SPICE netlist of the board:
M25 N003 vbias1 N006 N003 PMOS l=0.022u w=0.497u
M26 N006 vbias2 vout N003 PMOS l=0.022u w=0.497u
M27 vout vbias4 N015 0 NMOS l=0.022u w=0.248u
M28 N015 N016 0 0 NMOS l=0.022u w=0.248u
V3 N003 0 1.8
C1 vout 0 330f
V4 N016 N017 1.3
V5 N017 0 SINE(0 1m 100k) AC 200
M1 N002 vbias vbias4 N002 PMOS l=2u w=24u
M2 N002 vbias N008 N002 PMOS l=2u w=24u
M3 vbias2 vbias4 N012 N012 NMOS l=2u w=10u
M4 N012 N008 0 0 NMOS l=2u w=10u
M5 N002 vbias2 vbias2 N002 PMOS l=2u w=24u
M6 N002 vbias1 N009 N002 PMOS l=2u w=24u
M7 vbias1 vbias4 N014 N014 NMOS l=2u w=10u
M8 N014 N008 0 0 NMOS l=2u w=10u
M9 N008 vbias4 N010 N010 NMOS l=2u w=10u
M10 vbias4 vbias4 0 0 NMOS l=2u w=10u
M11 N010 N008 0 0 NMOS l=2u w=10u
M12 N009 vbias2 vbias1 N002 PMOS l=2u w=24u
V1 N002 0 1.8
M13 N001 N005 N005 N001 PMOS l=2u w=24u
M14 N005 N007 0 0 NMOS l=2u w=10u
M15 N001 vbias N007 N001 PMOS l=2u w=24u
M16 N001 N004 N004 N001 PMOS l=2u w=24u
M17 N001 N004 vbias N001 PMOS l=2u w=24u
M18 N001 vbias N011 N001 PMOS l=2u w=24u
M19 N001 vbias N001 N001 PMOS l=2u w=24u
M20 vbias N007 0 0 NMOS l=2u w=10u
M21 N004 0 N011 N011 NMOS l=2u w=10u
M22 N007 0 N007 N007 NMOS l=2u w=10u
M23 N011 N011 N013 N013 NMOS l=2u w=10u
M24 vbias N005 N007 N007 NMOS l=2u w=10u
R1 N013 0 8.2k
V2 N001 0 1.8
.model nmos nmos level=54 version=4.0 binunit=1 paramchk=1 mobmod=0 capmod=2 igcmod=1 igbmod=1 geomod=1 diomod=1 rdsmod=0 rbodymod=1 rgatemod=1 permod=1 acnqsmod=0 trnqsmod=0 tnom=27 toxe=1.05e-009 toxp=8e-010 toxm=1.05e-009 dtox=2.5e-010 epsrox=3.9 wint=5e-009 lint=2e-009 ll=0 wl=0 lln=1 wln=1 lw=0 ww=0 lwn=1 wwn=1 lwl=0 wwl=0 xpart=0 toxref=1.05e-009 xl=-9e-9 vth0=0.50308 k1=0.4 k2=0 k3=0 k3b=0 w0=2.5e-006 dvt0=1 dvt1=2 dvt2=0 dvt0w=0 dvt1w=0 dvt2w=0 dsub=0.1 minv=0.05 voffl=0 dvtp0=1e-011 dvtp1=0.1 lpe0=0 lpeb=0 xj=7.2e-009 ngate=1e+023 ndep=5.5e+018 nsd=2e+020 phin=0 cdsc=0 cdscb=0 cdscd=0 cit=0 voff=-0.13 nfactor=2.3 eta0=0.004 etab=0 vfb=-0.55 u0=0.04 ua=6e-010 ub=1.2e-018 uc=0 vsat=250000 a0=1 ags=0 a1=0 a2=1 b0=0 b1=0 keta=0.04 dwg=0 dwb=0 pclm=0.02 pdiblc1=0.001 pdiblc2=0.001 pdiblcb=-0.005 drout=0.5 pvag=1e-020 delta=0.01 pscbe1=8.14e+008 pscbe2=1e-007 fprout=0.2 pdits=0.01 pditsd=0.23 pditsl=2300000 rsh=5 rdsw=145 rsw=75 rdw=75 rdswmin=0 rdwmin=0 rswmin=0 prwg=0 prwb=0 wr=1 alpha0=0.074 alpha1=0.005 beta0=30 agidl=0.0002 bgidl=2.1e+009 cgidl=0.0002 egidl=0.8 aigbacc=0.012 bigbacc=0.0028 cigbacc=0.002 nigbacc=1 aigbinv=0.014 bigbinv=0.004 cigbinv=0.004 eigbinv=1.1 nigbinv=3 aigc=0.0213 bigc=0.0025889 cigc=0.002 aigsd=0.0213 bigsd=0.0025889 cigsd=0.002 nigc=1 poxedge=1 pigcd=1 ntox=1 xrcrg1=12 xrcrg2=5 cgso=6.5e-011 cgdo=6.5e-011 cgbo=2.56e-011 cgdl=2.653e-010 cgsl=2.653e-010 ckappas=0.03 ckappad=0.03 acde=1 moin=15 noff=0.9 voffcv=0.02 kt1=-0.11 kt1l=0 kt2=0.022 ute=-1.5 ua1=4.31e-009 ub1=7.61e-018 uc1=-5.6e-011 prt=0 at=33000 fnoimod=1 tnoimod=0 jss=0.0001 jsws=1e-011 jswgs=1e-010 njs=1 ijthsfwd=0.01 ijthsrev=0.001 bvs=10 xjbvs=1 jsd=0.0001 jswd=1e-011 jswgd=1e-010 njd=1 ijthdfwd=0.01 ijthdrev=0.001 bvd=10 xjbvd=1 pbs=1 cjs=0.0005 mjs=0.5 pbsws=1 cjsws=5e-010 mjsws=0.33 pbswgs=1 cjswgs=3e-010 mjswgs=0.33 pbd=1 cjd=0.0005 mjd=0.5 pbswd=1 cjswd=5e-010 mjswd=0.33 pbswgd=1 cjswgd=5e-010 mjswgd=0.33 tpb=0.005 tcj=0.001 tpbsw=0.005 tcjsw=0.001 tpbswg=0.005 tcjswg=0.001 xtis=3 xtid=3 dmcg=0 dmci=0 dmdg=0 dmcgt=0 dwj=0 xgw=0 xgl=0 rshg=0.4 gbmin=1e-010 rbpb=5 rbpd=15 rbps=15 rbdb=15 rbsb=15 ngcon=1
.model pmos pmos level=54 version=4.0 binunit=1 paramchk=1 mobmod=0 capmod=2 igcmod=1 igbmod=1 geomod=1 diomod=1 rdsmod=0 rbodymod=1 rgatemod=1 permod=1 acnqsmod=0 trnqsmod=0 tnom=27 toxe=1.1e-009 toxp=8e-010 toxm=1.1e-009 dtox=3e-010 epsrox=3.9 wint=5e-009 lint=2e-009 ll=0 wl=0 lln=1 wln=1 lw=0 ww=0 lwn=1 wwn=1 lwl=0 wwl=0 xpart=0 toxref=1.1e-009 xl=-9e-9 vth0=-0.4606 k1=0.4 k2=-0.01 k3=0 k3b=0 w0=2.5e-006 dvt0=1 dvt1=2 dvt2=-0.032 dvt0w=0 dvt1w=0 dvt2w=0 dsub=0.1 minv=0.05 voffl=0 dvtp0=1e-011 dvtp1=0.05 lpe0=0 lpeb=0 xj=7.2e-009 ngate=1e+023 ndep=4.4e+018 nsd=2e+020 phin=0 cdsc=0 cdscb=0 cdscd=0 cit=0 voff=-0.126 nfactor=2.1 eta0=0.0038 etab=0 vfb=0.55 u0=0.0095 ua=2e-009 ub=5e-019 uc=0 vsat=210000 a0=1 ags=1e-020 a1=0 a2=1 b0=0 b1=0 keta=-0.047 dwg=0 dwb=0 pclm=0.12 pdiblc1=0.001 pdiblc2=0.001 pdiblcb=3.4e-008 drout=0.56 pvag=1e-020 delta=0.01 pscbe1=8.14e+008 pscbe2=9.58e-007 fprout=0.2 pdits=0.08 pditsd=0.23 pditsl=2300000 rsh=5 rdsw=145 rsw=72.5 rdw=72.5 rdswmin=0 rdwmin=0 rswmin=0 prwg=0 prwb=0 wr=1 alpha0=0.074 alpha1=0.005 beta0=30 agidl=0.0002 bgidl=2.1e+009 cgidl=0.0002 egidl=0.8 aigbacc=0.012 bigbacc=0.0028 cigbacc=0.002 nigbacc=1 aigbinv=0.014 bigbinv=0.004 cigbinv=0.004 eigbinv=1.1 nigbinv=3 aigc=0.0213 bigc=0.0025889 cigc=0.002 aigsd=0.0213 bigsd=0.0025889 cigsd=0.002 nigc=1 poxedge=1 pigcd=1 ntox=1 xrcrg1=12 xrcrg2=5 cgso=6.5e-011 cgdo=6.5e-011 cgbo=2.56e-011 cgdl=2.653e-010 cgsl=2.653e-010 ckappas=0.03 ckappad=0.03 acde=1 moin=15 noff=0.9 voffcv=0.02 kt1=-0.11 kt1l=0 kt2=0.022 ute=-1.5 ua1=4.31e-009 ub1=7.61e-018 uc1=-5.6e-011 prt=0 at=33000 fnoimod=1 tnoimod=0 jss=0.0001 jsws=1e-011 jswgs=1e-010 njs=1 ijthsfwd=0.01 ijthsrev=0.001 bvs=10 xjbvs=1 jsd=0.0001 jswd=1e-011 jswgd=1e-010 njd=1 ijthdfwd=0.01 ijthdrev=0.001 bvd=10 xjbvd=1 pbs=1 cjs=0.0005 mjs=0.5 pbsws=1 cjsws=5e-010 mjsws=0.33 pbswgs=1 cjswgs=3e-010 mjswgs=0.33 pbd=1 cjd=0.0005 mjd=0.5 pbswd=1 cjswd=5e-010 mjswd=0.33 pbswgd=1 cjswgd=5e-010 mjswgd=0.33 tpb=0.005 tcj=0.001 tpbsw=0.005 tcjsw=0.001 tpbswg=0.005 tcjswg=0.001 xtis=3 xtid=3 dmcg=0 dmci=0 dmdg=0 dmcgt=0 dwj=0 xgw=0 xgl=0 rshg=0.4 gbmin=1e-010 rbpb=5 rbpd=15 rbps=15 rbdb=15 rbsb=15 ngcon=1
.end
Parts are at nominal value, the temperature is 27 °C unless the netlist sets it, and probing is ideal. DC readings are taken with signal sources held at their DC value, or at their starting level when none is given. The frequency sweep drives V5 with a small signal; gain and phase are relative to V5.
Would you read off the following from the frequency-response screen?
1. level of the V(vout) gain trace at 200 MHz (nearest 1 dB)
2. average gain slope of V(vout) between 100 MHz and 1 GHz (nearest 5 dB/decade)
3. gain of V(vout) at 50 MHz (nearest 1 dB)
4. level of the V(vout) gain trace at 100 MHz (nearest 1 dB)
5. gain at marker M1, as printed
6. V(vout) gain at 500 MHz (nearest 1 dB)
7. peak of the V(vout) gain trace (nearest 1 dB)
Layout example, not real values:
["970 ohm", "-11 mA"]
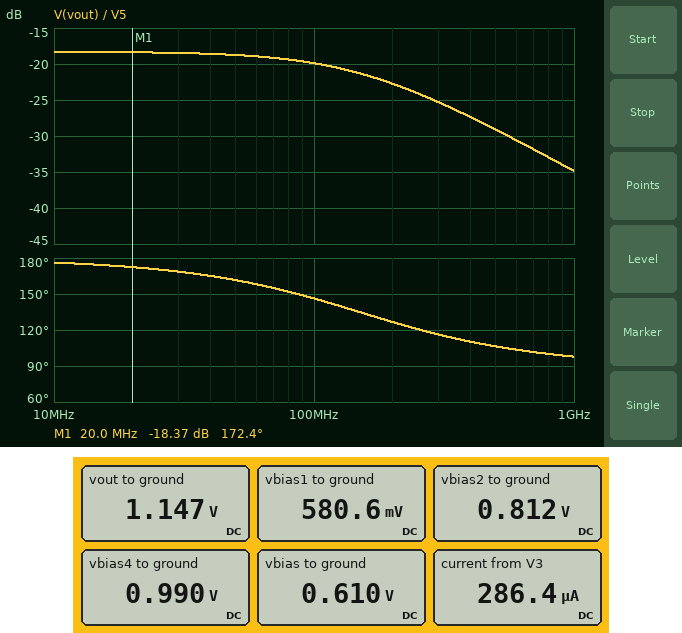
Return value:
["-23 dB", "-15 dB/decade", "-19 dB", "-20 dB", "-18.37 dB", "-29 dB", "-18 dB"]
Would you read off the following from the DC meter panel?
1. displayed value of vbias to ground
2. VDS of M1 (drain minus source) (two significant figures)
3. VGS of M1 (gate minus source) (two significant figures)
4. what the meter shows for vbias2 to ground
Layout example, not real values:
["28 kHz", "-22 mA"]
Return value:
["0.610 V", "810 mV", "-380 mV", "0.812 V"]
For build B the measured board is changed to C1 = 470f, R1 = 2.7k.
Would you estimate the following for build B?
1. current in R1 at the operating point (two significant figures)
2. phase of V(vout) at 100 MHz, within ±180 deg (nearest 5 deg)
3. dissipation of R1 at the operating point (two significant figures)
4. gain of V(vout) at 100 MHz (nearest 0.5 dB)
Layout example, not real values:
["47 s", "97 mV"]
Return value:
["63 µA", "135 deg", "11 µW", "-21.0 dB"]
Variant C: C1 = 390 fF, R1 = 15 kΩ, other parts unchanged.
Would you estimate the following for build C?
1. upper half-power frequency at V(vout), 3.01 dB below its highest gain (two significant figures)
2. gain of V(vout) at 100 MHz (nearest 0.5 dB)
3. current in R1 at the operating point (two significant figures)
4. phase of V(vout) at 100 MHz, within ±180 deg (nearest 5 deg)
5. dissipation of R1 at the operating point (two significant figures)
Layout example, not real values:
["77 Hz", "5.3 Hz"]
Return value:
["130 MHz", "-20.5 dB", "21 µA", "140 deg", "6.8 µW"]
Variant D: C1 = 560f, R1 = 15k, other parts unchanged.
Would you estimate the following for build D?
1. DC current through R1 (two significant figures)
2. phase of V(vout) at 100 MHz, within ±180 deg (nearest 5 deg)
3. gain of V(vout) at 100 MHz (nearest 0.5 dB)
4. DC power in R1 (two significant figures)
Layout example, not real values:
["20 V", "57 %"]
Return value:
["21 µA", "130 deg", "-22.0 dB", "6.8 µW"]
